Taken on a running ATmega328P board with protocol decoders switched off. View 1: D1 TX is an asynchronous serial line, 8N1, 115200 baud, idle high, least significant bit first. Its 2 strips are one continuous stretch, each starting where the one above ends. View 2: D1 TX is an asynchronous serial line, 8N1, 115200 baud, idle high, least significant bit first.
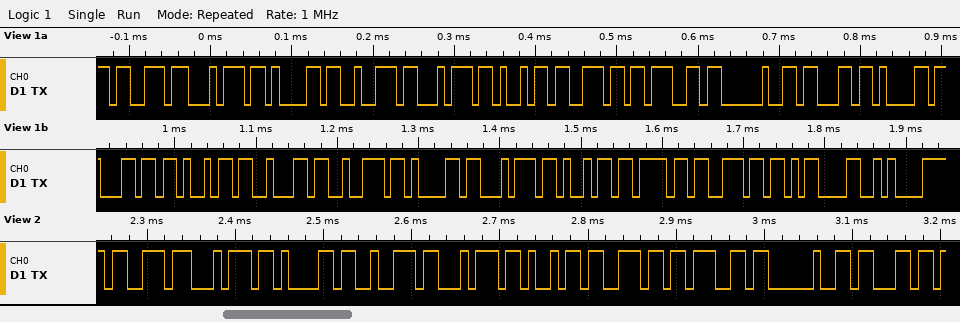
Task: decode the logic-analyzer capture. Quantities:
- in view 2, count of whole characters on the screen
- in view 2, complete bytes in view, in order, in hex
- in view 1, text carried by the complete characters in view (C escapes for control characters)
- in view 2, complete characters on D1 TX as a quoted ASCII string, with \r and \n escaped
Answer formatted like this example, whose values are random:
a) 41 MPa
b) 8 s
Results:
a) 10
b) 73 74 61 72 74 69 6E 67 20 63
c) "starting calibration\r\n"
d) "starting c"
